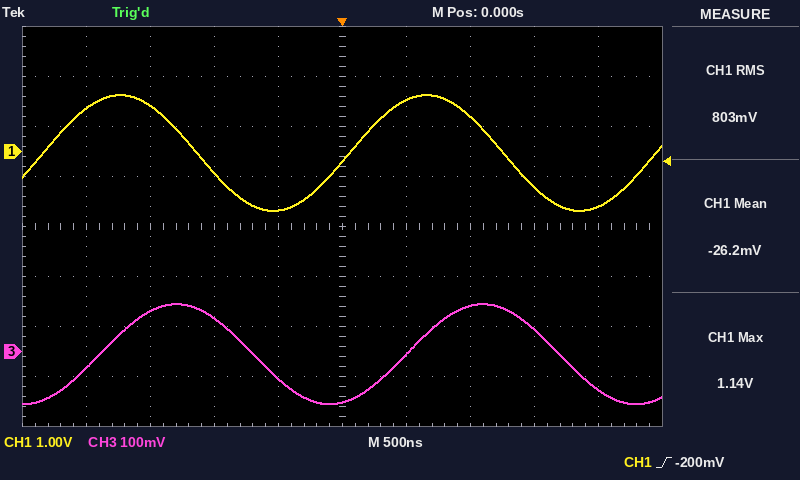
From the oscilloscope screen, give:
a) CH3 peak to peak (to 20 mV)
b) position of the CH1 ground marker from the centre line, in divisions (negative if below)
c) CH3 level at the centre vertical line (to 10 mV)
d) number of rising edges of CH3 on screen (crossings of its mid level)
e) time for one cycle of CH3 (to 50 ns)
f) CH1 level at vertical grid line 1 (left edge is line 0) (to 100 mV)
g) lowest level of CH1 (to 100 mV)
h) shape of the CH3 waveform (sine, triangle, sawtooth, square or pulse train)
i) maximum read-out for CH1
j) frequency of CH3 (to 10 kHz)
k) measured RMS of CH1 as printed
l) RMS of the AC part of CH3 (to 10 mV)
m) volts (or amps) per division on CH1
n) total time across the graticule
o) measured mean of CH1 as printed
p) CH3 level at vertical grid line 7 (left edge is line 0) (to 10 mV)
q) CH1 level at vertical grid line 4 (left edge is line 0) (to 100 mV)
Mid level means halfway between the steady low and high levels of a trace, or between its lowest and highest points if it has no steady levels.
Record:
200 mV
+1.5 div
-100 mV
2
2.40 µs
900 mV
-1.2 V
sine
1.14 V
420 kHz
803 mV
70 mV
1 V
5 µs
-26.2 mV
90 mV
-1.2 V
